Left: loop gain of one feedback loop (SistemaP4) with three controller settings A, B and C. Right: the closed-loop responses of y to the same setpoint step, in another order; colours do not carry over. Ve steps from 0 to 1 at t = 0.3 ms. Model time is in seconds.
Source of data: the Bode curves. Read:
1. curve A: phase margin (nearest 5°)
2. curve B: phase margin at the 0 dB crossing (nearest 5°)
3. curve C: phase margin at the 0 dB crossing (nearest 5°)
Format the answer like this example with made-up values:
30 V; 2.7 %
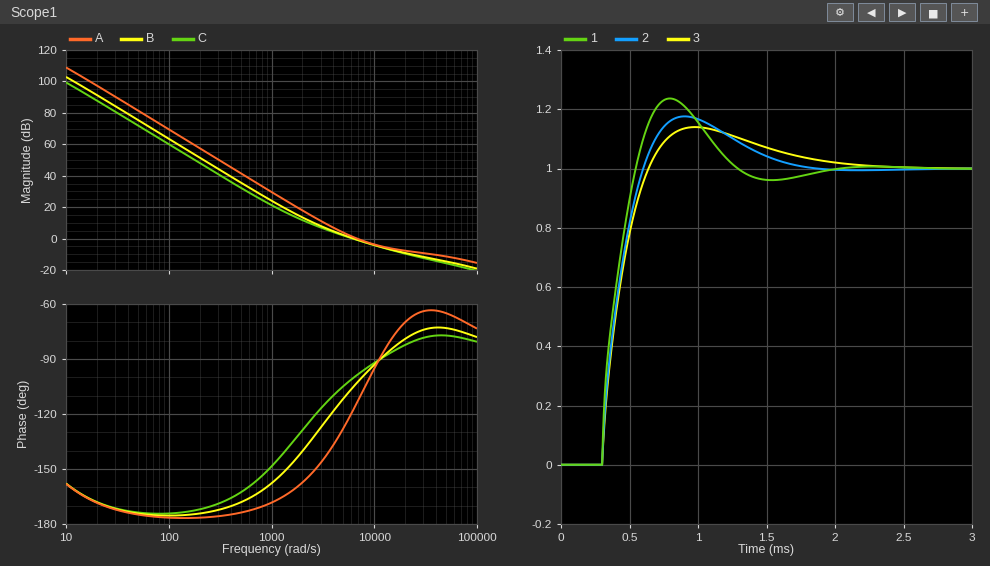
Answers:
65°; 75°; 80°
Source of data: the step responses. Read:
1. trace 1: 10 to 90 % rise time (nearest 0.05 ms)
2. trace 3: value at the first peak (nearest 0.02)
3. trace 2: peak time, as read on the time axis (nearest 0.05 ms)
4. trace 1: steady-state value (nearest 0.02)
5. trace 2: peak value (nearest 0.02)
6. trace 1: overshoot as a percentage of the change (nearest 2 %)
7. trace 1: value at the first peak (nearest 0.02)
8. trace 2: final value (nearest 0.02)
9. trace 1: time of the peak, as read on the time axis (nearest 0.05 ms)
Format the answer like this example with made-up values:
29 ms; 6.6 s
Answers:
0.20 ms; 1.14; 0.90 ms; 1.00; 1.18; 24 %; 1.24; 1.00; 0.80 ms
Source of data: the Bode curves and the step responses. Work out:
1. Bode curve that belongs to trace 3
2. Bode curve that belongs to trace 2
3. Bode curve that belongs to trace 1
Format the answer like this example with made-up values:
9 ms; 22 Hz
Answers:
C; B; A
